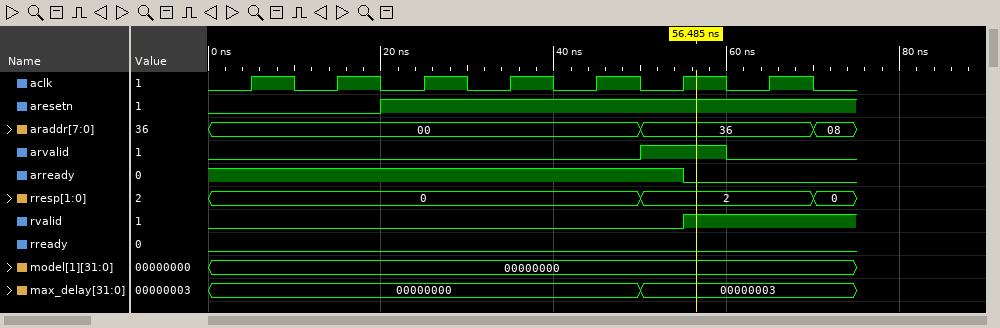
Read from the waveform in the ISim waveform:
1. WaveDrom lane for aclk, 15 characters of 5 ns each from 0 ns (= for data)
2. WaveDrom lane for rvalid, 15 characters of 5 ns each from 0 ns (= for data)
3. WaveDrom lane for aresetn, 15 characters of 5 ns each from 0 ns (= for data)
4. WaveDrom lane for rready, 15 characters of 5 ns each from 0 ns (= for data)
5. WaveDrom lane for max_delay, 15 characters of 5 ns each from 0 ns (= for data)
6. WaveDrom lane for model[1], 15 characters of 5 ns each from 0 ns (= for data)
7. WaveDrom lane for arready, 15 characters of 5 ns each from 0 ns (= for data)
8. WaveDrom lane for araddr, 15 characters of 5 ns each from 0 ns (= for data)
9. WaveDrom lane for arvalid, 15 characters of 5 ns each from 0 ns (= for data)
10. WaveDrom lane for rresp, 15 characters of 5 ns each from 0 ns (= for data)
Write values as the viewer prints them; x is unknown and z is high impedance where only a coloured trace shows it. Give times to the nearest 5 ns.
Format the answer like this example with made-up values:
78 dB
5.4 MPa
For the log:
{name: 'aclk', wave: '010101010101010'}
{name: 'rvalid', wave: '0..........1...'}
{name: 'aresetn', wave: '0...1..........'}
{name: 'rready', wave: '0..............'}
{name: 'max_delay', wave: '=.........=....', data: '00000000 00000003'}
{name: 'model[1]', wave: '=..............', data: '00000000'}
{name: 'arready', wave: '1..........0...'}
{name: 'araddr', wave: '=.........=...=', data: '00 36 08'}
{name: 'arvalid', wave: '0.........1.0..'}
{name: 'rresp', wave: '=.........=...=', data: '0 2 0'}
